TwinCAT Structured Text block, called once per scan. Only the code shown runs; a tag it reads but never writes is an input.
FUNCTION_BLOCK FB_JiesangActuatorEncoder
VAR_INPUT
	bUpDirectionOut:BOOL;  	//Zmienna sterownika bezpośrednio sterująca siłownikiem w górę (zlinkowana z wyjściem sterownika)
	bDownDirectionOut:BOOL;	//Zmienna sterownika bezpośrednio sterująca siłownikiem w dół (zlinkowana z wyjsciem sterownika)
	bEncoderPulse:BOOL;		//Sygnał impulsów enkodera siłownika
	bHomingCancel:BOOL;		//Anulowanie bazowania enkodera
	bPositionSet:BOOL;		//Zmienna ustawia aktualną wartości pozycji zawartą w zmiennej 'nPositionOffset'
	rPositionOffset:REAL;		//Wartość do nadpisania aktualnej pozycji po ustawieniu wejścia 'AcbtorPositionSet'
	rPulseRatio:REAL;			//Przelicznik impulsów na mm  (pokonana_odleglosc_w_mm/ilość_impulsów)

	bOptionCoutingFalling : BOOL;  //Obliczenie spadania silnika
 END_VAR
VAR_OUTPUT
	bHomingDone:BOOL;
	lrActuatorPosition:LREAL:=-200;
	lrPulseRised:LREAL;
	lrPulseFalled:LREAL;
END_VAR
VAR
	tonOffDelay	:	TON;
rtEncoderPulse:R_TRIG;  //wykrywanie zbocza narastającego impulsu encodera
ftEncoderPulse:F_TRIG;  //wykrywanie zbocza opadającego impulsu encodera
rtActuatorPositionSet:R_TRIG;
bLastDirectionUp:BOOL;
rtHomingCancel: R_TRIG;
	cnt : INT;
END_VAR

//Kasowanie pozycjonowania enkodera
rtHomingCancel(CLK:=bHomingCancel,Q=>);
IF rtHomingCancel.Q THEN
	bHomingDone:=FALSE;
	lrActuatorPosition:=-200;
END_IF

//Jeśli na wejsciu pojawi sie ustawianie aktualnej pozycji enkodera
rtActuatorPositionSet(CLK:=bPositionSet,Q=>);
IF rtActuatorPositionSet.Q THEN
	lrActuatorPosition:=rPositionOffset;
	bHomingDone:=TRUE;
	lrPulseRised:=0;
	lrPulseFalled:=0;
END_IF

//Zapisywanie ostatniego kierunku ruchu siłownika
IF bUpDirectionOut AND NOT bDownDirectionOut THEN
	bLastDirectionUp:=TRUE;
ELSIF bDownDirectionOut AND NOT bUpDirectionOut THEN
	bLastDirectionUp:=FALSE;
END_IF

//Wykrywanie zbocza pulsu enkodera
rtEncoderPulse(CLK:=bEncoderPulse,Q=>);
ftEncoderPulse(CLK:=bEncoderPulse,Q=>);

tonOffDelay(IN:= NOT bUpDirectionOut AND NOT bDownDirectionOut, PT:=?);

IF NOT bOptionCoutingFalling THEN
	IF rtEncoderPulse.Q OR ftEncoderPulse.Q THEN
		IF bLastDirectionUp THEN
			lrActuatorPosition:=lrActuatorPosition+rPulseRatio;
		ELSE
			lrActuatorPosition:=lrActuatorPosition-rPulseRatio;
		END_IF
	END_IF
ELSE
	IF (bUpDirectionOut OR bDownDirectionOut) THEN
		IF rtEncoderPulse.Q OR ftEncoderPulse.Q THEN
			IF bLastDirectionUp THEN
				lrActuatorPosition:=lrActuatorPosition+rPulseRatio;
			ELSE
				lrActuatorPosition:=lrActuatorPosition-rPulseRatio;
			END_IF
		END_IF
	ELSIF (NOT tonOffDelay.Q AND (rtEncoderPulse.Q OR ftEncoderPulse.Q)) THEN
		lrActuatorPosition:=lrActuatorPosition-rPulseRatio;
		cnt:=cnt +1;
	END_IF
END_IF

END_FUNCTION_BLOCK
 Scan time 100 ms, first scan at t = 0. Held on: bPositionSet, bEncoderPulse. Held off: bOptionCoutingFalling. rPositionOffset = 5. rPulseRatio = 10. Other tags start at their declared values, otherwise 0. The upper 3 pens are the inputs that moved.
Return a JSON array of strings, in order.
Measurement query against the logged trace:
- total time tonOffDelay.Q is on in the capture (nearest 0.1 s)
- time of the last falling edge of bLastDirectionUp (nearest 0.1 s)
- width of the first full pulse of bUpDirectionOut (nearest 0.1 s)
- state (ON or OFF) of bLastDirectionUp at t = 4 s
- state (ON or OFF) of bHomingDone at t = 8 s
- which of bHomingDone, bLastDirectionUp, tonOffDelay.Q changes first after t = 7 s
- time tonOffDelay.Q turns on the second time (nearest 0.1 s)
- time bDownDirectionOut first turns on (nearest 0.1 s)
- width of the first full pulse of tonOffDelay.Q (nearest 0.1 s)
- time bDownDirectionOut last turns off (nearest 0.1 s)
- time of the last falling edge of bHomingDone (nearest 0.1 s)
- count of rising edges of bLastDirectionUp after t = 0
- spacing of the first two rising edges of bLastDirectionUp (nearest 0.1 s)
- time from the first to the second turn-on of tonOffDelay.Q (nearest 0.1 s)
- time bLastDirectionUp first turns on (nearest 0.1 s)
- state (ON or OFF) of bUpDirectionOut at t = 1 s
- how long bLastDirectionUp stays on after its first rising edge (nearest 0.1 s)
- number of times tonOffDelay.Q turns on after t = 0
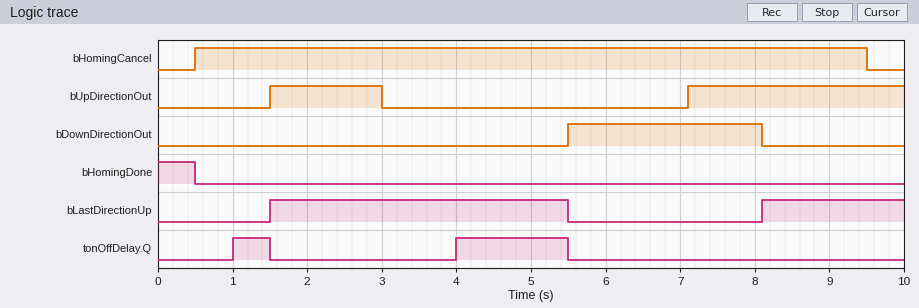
["2.0 s", "5.5 s", "1.5 s", "ON", "OFF", "bLastDirectionUp", "4.0 s", "5.5 s", "0.5 s", "8.1 s", "0.5 s", "2", "6.6 s", "3.0 s", "1.5 s", "OFF", "4.0 s", "2"]
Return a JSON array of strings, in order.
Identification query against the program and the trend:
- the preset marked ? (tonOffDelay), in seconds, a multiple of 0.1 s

["1.0 s"]
